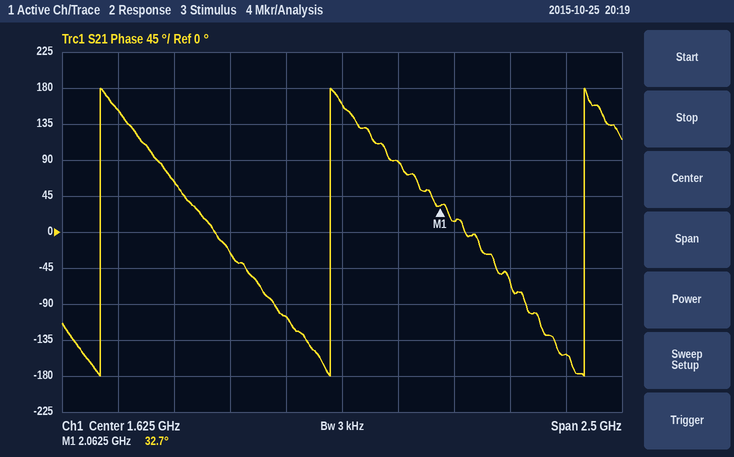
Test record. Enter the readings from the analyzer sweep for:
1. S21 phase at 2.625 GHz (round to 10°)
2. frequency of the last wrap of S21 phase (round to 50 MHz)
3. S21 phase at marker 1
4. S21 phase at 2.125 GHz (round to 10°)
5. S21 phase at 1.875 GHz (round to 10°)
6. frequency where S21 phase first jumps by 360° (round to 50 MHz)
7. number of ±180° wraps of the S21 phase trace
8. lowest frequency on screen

-150°
2.70 GHz
32.7°
10°
90°
550 MHz
3
375 MHz
